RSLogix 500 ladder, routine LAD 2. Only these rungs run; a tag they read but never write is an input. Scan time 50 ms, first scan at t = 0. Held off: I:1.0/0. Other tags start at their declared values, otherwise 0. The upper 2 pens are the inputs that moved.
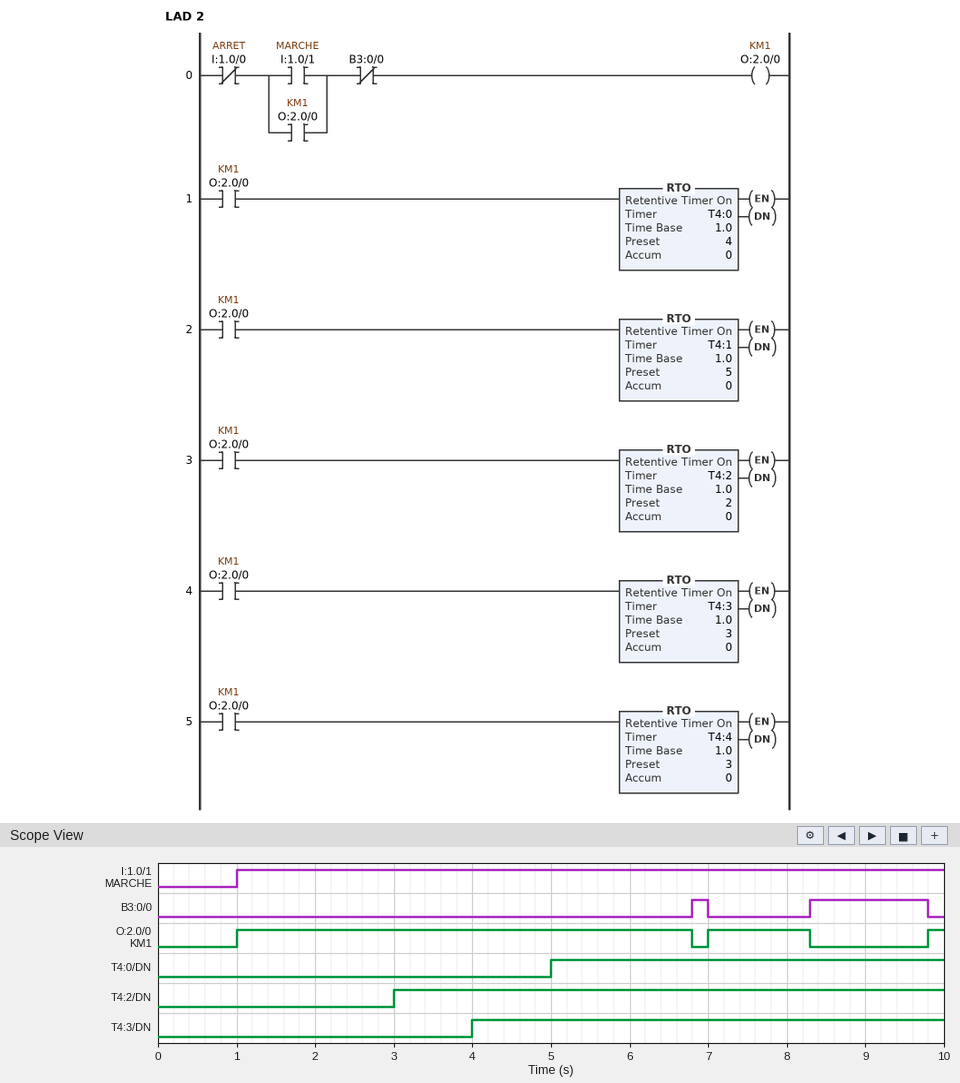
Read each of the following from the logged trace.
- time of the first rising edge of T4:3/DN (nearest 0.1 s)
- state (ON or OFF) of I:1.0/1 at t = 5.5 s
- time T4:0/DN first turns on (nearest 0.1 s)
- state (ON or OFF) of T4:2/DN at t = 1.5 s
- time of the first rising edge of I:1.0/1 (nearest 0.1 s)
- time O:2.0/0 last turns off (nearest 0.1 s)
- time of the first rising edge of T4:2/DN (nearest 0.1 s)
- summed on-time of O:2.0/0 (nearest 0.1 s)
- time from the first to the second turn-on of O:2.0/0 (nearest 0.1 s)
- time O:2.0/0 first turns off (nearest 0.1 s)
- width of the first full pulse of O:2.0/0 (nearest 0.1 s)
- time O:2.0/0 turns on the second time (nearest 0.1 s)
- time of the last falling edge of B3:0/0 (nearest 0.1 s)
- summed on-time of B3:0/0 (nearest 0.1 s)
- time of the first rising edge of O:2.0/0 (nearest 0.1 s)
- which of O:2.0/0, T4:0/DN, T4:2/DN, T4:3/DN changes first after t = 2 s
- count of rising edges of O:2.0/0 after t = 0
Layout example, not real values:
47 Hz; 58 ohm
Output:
4.0 s; ON; 5.0 s; OFF; 1.0 s; 8.3 s; 3.0 s; 7.3 s; 6.0 s; 6.8 s; 5.8 s; 7.0 s; 9.8 s; 1.7 s; 1.0 s; T4:2/DN; 3
